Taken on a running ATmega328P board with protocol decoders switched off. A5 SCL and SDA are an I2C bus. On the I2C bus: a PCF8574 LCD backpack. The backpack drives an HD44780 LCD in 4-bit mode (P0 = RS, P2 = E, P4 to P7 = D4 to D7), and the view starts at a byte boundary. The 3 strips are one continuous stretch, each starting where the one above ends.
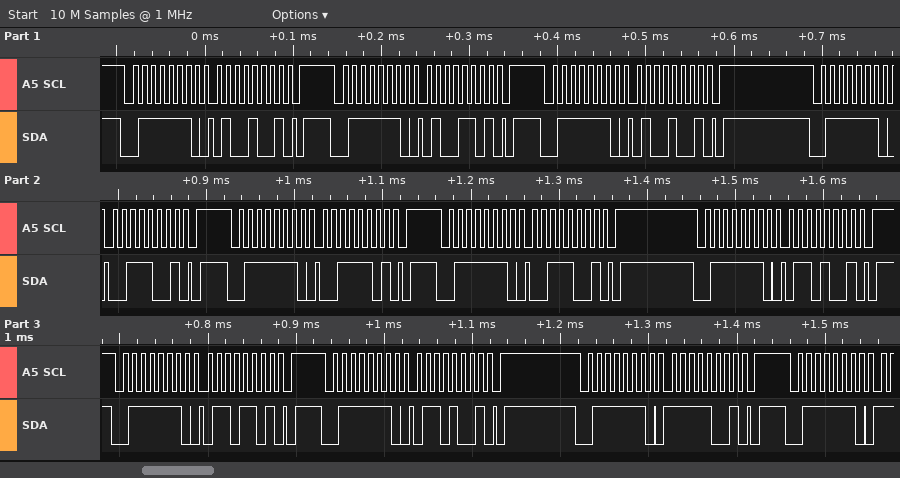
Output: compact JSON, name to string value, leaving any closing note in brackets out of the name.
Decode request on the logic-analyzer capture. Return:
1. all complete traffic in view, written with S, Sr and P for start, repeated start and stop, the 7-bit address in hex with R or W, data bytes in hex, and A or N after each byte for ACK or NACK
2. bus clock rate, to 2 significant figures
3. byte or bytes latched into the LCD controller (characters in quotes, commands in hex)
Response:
{"all complete traffic in view, written with S, Sr and P for start, repeated start and stop, the 7-bit address in hex with R or W, data bytes in hex, and A or N after each byte for ACK or NACK": "S 3FW A 49 A P S 3FW A 4D A P S 3FW A 49 A P S 3FW A 39 A P S 3FW A 3D A P S 3FW A 39 A P S 3FW A 69 A P S 3FW A 6D A P S 3FW A 69 A P S 3FW A F9 A P S 3FW A", "bus clock rate, to 2 significant figures": "100 kHz", "byte or bytes latched into the LCD controller": "'C'"}
